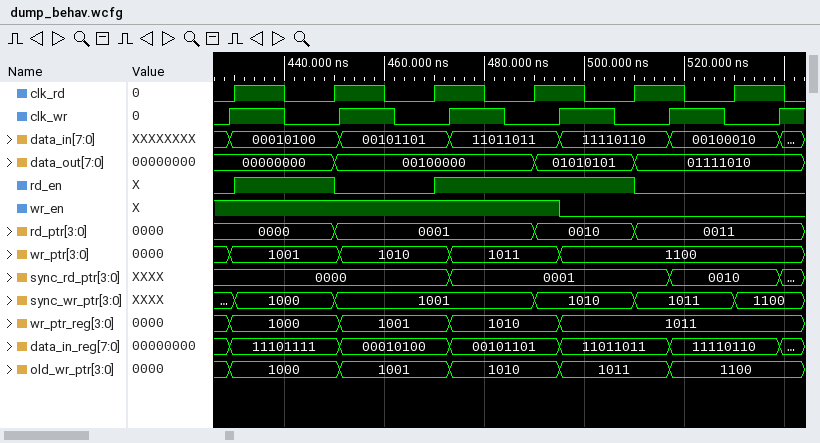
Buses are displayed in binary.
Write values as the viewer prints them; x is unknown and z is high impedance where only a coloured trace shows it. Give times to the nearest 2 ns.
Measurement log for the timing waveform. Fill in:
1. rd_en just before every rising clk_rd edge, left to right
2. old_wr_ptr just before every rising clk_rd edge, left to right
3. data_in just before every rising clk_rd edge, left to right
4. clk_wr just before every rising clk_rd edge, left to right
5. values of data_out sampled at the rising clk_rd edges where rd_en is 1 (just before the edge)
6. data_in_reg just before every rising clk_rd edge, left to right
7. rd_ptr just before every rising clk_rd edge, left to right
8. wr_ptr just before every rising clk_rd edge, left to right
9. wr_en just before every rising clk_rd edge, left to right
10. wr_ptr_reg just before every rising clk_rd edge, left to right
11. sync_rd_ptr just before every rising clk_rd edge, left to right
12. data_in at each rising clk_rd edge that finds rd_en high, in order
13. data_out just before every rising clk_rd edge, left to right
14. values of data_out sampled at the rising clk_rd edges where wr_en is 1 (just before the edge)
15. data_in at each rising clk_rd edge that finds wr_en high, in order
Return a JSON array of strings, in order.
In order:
["0 1 0 1 1 0", "1000, 1000, 1001, 1010, 1011, 1100", "00010100, 00010100, 00101101, 11011011, 11110110, 00100010", "1 0 0 0 0 0", "00000000, 00100000, 01010101", "11101111, 11101111, 00010100, 00101101, 11011011, 11110110", "0000, 0000, 0001, 0001, 0010, 0011", "1001, 1001, 1010, 1011, 1100, 1100", "1 1 1 1 0 0", "1000, 1000, 1001, 1010, 1011, 1011", "0000, 0000, 0000, 0001, 0001, 0010", "00010100, 11011011, 11110110", "00000000, 00000000, 00100000, 00100000, 01010101, 01111010", "00000000, 00000000, 00100000, 00100000", "00010100, 00010100, 00101101, 11011011"]
